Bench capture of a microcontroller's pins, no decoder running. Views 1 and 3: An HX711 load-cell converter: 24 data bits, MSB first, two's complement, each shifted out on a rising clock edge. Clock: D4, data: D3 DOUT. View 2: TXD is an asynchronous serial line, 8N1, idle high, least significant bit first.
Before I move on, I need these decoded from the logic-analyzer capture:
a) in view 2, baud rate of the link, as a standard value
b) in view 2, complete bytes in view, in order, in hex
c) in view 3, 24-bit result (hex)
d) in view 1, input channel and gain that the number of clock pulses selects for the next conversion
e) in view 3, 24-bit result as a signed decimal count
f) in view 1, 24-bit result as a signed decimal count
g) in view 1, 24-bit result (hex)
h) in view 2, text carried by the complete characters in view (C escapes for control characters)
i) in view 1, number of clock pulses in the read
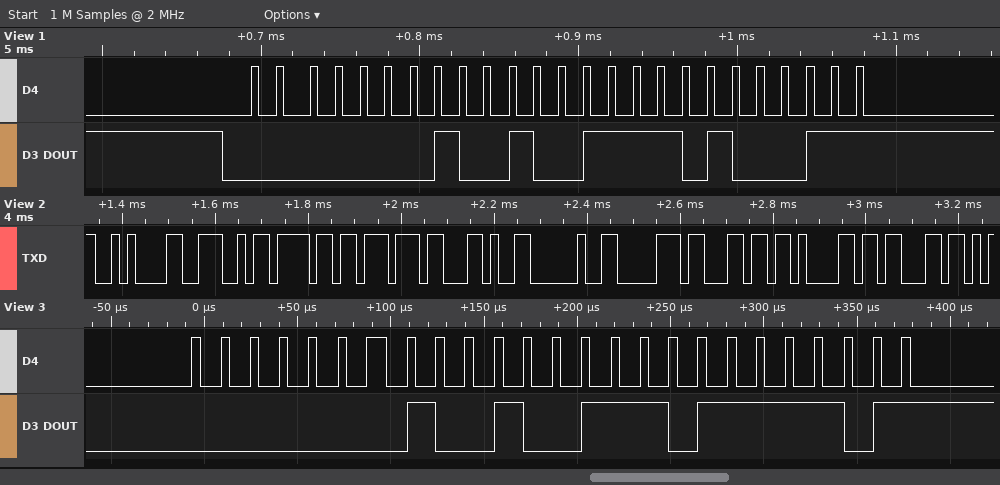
57600 baud
0A 4E 6F 77 2C 20 70 6C 61 63
0x01277D
channel A, gain 128
75645
75683
0x0127A3
"\nNow, plac"
25
